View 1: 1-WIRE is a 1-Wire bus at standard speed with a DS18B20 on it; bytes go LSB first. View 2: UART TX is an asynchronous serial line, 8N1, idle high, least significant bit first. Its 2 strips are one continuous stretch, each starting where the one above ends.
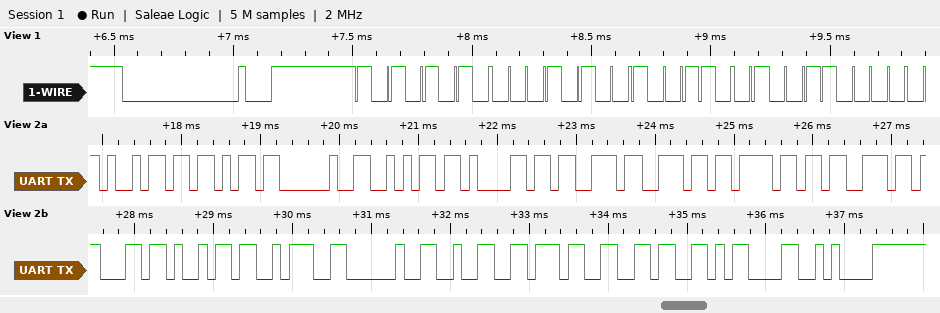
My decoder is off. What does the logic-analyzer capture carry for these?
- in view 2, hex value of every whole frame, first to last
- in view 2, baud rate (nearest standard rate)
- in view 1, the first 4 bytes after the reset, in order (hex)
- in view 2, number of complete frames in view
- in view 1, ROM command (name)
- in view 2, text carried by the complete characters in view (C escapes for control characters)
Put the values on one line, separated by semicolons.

69 6B 20 6A 61 73 6E 6F 73 63 69 3A 20 32 37 36 0D 0A; 9600 baud; 55 28 99 0C; 18; Match ROM; "ik jasnosci: 276\r\n"
